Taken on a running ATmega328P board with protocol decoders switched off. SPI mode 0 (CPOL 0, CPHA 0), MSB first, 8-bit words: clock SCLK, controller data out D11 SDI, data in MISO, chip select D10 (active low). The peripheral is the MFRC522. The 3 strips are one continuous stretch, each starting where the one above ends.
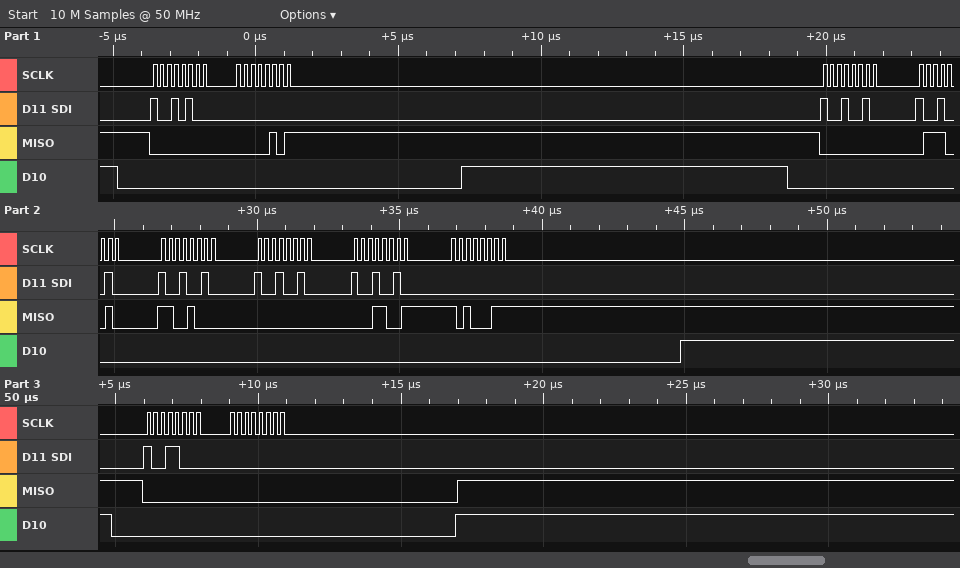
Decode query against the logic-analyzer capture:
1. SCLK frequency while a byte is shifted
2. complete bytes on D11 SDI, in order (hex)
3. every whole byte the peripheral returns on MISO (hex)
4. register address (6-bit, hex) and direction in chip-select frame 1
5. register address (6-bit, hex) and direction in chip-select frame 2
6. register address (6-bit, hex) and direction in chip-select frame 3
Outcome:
4 MHz
0x94 0x00 0x92 0x92 0x92 0x92 0x92 0x00 0x98 0x00
0x00 0x05 0x00 0x72 0xC8 0x00 0x19 0xA3 0x00 0x00
0x0A read
0x09 read
0x0C read
